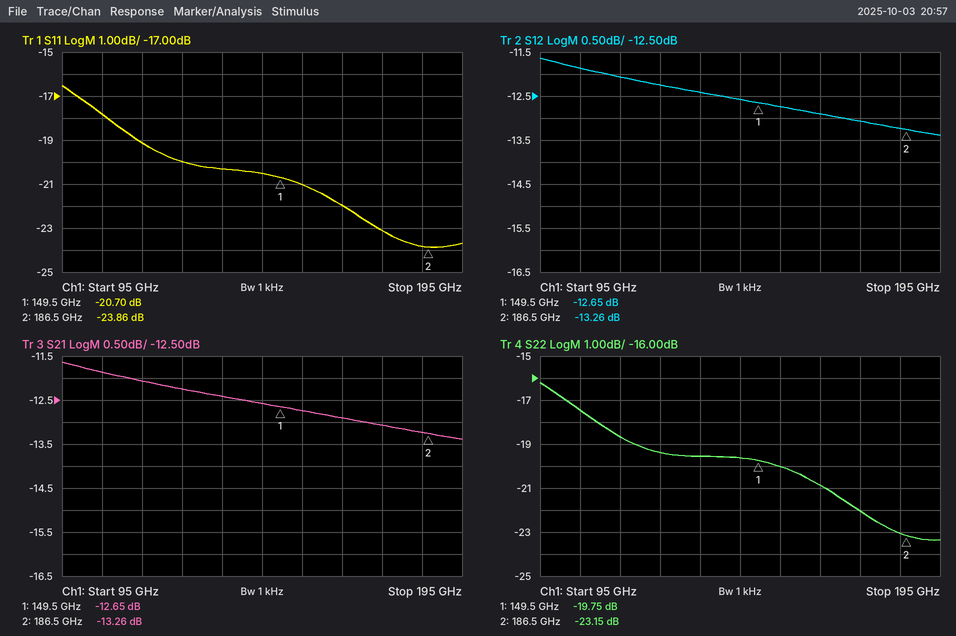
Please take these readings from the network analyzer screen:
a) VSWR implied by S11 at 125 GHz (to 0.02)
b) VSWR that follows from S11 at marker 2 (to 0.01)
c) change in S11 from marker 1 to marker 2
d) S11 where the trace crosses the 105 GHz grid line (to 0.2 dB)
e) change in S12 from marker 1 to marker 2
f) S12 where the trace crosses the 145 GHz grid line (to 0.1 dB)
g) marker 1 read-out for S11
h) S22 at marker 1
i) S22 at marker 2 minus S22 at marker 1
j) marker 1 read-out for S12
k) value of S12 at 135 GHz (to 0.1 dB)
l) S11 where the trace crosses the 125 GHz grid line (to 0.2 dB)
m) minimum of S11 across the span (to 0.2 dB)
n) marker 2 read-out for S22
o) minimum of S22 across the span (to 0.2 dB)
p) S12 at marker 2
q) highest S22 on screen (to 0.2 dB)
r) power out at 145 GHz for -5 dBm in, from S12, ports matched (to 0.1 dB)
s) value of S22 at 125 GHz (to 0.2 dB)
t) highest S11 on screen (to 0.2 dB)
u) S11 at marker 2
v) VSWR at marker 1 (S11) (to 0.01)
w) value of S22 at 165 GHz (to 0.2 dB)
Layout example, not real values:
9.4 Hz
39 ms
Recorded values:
1.22
1.14
-3.16 dB
-17.8 dB
-0.61 dB
-12.6 dB
-20.70 dB
-19.75 dB
-3.40 dB
-12.65 dB
-12.4 dB
-20.0 dB
-23.8 dB
-23.15 dB
-23.4 dB
-13.26 dB
-16.2 dB
-17.6 dBm
-19.4 dB
-16.6 dB
-23.86 dB
1.20
-20.8 dB
